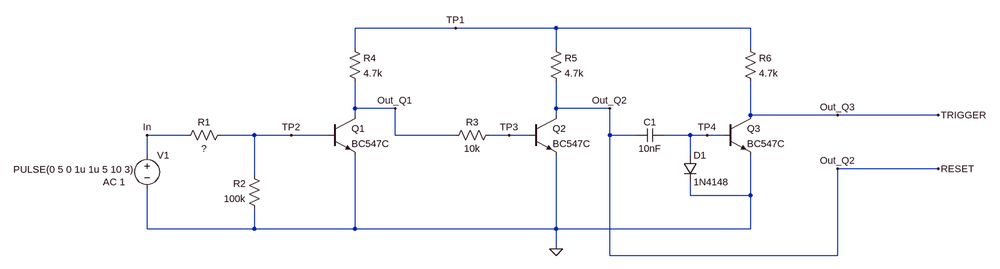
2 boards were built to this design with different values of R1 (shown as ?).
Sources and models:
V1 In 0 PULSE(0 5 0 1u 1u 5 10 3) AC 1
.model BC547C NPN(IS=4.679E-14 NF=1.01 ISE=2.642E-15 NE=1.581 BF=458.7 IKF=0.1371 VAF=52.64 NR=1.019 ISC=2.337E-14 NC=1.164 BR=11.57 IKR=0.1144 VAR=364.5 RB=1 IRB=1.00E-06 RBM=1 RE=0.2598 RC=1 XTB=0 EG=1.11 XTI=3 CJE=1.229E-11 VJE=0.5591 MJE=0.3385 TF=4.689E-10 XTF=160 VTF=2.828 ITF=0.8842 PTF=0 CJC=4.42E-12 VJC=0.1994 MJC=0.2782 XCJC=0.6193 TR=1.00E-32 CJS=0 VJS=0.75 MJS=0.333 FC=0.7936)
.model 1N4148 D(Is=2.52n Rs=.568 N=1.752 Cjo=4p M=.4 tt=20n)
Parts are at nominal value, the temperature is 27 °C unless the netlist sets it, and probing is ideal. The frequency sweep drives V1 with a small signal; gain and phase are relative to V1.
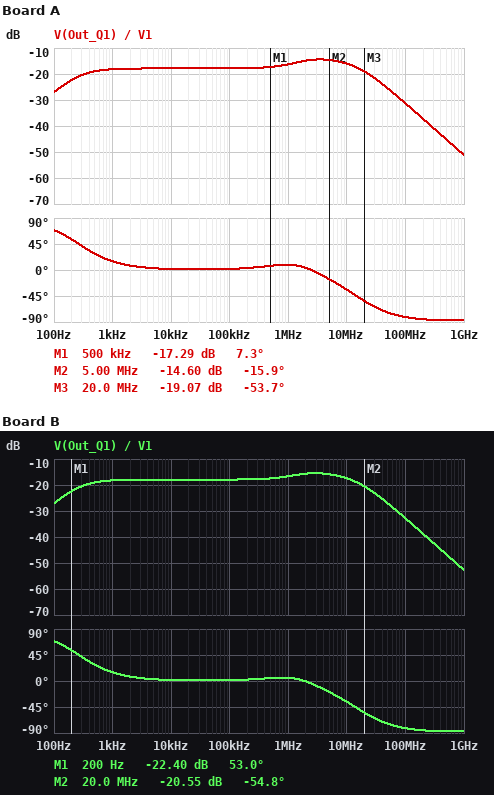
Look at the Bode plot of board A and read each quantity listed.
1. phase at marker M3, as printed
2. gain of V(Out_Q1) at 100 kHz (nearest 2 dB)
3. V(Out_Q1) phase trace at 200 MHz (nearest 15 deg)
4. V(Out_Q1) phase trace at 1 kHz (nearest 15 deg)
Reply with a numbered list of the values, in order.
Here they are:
1. -53.7 deg
2. -18 dB
3. -90 deg
4. 15 deg
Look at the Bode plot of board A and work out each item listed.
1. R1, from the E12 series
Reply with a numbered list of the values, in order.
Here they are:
1. 4.7 kΩ
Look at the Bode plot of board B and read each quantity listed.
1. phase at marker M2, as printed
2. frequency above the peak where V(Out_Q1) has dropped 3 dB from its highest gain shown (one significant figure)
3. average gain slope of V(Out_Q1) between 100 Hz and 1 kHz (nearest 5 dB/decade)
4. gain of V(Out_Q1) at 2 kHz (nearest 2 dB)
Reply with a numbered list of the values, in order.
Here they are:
1. -54.8 deg
2. 10 MHz
3. 10 dB/decade
4. -18 dB
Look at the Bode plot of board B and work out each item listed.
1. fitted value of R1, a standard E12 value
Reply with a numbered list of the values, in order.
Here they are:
1. 5.6 kΩ
